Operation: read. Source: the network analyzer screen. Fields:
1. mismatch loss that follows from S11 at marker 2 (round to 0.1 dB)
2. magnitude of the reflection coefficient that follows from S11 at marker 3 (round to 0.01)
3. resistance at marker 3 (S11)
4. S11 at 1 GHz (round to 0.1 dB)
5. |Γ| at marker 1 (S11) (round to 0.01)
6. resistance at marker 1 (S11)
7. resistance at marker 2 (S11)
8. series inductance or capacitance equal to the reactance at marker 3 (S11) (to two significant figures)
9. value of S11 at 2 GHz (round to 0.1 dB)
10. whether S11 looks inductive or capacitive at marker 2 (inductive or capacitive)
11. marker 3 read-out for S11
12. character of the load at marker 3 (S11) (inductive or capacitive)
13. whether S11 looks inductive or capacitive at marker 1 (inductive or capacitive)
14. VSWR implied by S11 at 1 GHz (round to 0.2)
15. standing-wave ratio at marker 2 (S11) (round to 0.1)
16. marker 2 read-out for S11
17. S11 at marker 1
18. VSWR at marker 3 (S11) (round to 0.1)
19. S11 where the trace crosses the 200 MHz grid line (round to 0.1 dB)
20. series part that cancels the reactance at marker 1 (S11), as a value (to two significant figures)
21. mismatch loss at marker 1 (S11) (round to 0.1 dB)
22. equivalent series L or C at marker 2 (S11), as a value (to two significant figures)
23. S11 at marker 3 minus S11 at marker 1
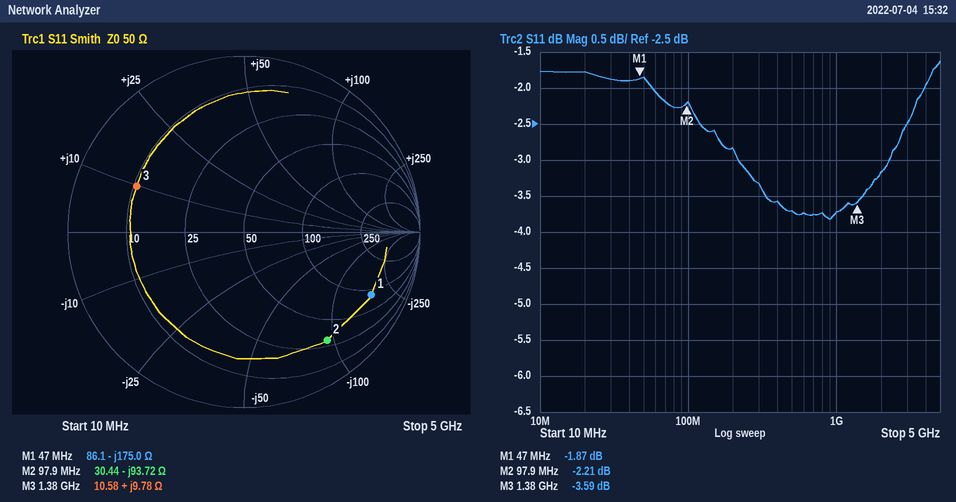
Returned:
4.0 dB
0.66
10.58 Ω
-3.7 dB
0.81
86.1 Ω
30.44 Ω
1.1 nH
-3.2 dB
capacitive
-3.59 dB
inductive
capacitive
4.8
7.9
-2.21 dB
-1.87 dB
4.9
-2.8 dB
590 nH
4.6 dB
17 pF
-1.72 dB
